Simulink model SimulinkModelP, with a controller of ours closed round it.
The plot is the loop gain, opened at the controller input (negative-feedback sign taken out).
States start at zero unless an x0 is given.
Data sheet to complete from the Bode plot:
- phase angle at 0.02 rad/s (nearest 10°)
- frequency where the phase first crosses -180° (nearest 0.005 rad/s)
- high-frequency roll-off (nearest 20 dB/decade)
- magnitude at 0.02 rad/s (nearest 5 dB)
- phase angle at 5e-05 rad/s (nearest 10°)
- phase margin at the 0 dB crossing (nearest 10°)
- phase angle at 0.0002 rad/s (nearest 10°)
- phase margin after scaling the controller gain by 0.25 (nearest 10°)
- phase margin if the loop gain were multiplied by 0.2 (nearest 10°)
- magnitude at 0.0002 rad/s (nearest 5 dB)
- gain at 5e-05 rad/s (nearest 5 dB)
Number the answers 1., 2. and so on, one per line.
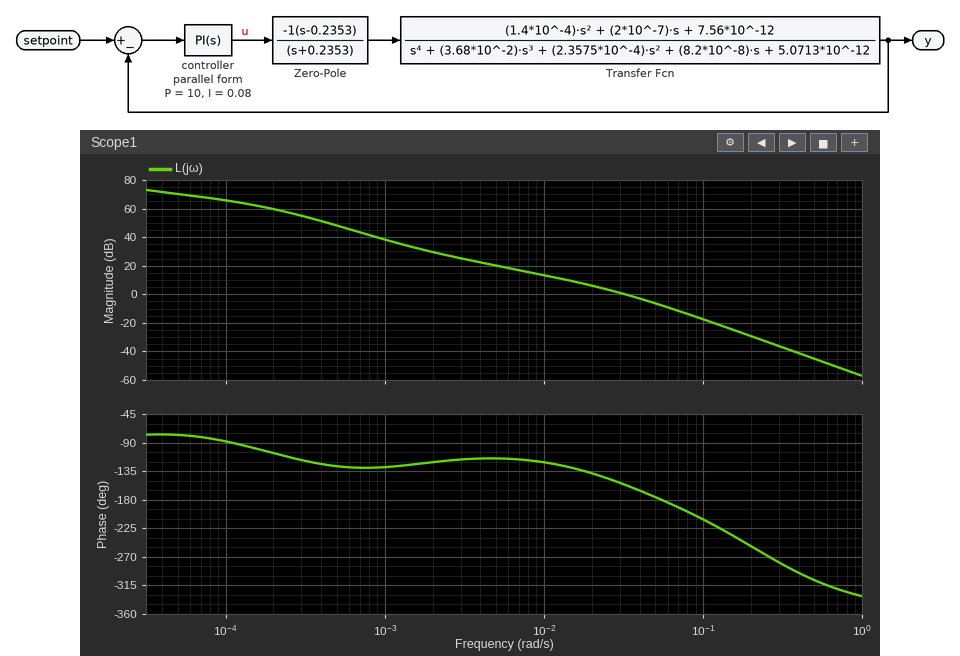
1. -140°
2. 0.055 rad/s
3. -40 dB/decade
4. 5 dB
5. -80°
6. 20°
7. -110°
8. 60°
9. 60°
10. 60 dB
11. 70 dB
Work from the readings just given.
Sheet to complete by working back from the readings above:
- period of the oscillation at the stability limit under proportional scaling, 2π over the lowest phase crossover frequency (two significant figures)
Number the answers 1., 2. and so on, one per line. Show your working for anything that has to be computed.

1. 2π / 0.055 = 110 s
